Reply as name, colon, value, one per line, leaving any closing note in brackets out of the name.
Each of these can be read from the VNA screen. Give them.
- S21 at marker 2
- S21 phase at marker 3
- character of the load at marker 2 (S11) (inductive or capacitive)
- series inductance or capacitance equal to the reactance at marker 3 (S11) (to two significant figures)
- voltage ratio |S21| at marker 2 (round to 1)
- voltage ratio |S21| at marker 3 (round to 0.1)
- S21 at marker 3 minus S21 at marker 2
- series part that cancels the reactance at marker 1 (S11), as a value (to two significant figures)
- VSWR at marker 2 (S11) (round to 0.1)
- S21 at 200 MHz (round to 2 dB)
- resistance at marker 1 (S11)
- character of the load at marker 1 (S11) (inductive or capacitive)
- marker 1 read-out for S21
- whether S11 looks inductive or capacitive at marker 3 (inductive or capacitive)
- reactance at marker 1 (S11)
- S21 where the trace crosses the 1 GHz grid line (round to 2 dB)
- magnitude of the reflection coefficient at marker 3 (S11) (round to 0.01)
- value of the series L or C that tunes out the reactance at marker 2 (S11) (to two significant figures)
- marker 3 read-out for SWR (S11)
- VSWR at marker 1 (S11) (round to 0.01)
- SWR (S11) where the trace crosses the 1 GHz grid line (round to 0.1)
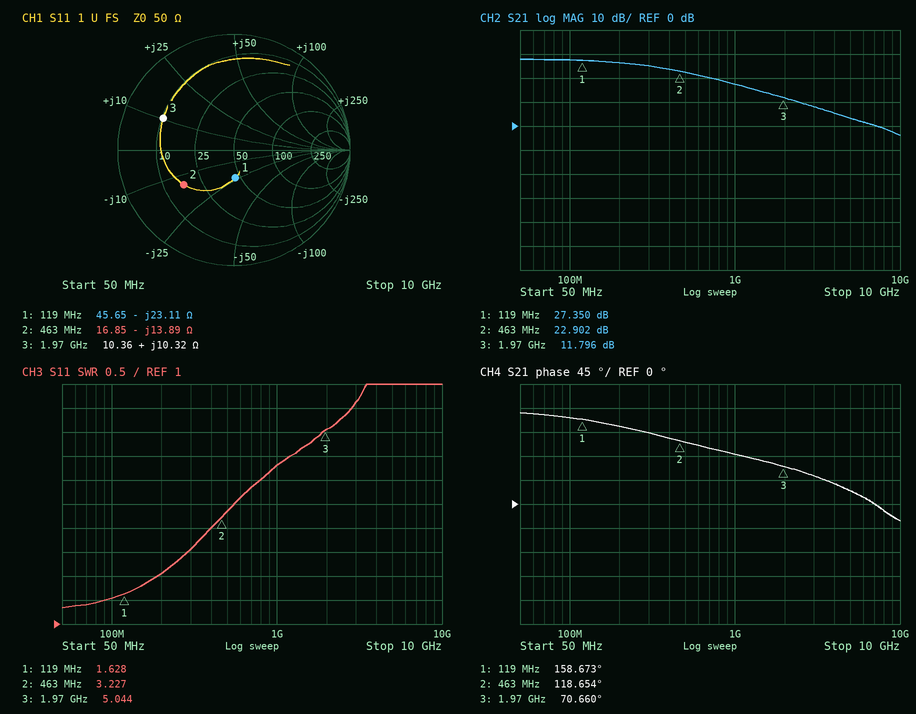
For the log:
S21 at marker 2: 22.902 dB
S21 phase at marker 3: 70.660°
character of the load at marker 2 (S11): capacitive
series inductance or capacitance equal to the reactance at marker 3 (S11): 830 pH
voltage ratio |S21| at marker 2: 14
voltage ratio |S21| at marker 3: 3.9
S21 at marker 3 minus S21 at marker 2: -11.106 dB
series part that cancels the reactance at marker 1 (S11), as a value: 31 nH
VSWR at marker 2 (S11): 3.2
S21 at 200 MHz: 26 dB
resistance at marker 1: 45.65 Ω
character of the load at marker 1 (S11): capacitive
marker 1 read-out for S21: 27.350 dB
whether S11 looks inductive or capacitive at marker 3: inductive
reactance at marker 1: -23.11 Ω
S21 where the trace crosses the 1 GHz grid line: 18 dB
magnitude of the reflection coefficient at marker 3 (S11): 0.67
value of the series L or C that tunes out the reactance at marker 2 (S11): 4.8 nH
marker 3 read-out for SWR: 5.044
VSWR at marker 1 (S11): 1.63
SWR (S11) where the trace crosses the 1 GHz grid line: 4.3
